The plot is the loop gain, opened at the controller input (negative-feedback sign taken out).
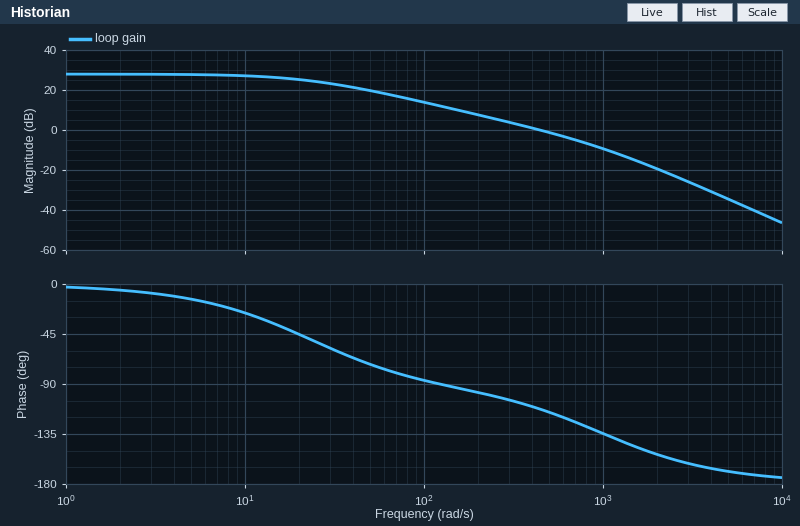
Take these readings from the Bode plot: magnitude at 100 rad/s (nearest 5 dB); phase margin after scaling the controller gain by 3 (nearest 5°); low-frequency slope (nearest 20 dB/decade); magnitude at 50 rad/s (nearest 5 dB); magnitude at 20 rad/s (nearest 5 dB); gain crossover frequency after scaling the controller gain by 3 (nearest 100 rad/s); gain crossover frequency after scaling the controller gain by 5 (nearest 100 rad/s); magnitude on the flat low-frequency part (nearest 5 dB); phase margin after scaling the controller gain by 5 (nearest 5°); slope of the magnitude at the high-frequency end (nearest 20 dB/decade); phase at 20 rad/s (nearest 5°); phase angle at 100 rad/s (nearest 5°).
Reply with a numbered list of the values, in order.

1. 15 dB
2. 45°
3. 0 dB/decade
4. 20 dB
5. 25 dB
6. 1000 rad/s
7. 1400 rad/s
8. 30 dB
9. 35°
10. -40 dB/decade
11. -45°
12. -85°
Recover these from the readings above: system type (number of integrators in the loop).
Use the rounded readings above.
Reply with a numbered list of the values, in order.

1. 0
